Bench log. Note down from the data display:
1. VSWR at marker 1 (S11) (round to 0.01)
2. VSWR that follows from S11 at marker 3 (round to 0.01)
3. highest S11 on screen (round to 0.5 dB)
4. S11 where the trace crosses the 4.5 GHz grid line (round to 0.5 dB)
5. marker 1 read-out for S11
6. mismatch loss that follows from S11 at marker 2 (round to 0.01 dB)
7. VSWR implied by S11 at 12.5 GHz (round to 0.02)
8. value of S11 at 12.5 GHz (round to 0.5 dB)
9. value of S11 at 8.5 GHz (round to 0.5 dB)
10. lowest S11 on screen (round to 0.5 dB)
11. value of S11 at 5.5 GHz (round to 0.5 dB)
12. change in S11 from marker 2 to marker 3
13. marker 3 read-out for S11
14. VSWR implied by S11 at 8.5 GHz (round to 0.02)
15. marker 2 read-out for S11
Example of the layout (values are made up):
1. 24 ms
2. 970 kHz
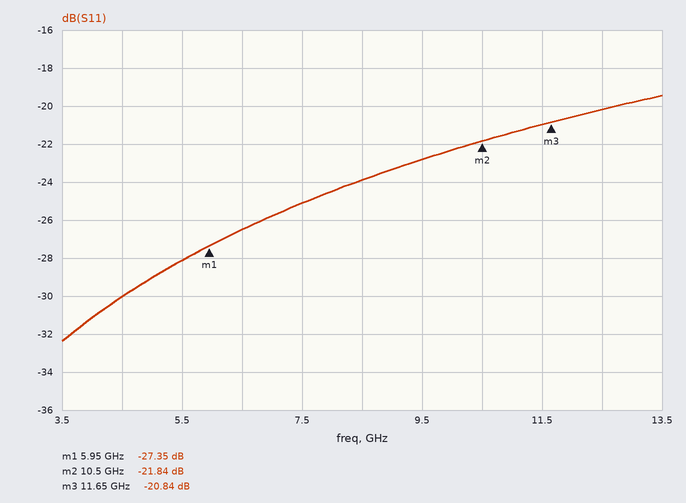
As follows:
1. 1.09
2. 1.20
3. -19.5 dB
4. -30.0 dB
5. -27.35 dB
6. 0.03 dB
7. 1.22
8. -20.0 dB
9. -24.0 dB
10. -32.5 dB
11. -28.0 dB
12. 1.00 dB
13. -20.84 dB
14. 1.14
15. -21.84 dB
